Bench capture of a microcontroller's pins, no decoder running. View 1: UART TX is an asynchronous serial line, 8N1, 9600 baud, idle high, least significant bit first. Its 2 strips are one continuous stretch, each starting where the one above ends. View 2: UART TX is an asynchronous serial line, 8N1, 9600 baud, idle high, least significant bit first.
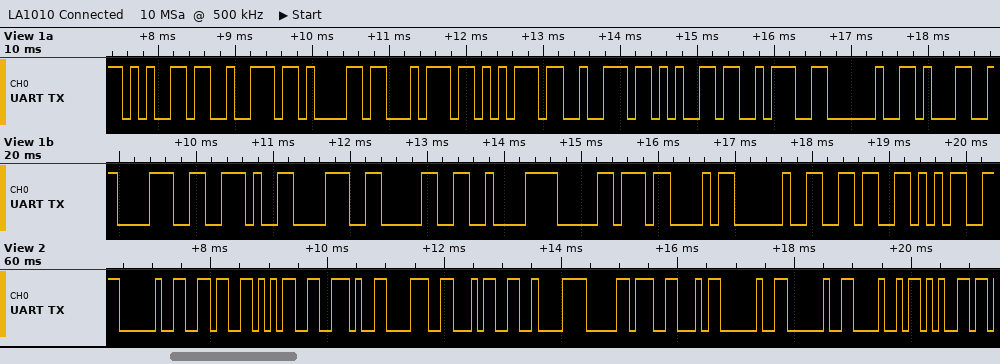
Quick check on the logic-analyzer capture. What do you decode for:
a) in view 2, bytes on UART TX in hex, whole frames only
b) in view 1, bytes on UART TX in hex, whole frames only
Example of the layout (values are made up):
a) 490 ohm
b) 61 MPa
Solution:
a) 20 36 35 2E 38 34 C2 B0 46 20 20 48 65
b) 65 72 61 74 75 72 65 3A 20 31 38 2E 38 30 C2 B0 43 20 36 35
